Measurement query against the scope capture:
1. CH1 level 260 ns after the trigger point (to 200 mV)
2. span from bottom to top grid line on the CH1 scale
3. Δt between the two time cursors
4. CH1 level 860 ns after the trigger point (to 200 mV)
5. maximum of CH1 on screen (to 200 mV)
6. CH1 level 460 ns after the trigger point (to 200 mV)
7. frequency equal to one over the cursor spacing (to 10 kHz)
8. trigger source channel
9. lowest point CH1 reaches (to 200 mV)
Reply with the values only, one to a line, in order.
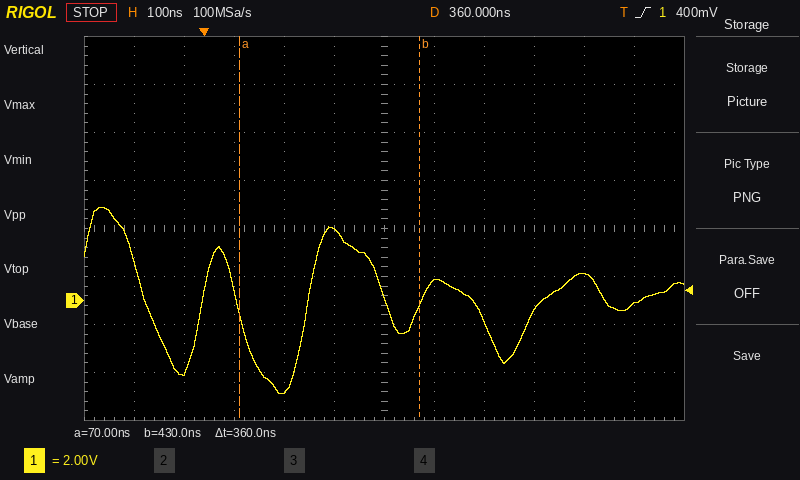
3.0 V
16 V
360 ns
-200 mV
3.8 V
800 mV
2.78 MHz
CH1
-3.8 V
